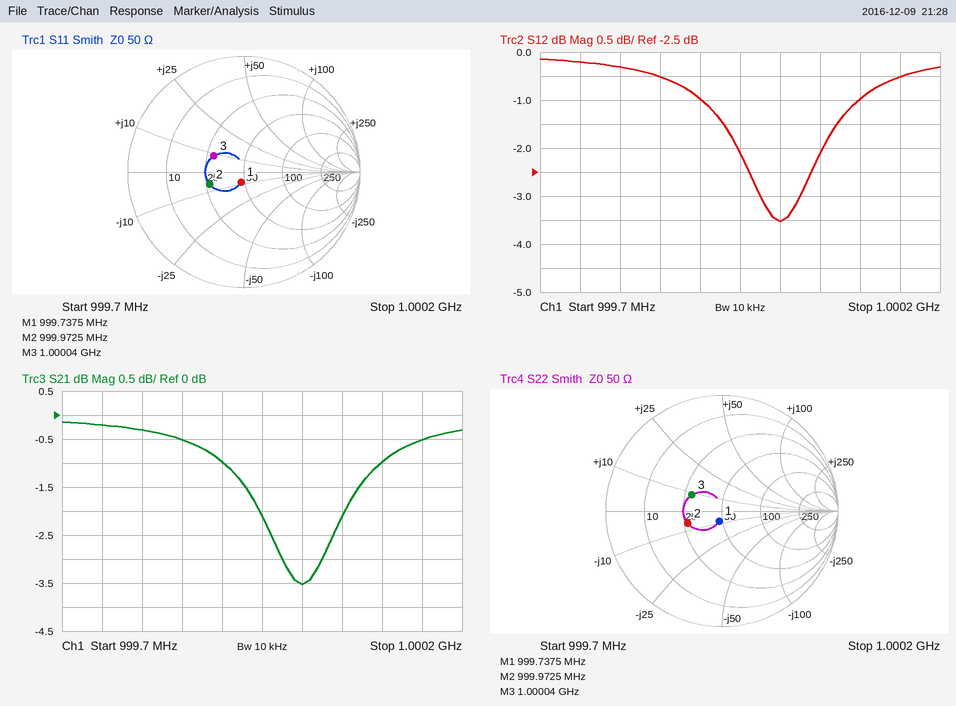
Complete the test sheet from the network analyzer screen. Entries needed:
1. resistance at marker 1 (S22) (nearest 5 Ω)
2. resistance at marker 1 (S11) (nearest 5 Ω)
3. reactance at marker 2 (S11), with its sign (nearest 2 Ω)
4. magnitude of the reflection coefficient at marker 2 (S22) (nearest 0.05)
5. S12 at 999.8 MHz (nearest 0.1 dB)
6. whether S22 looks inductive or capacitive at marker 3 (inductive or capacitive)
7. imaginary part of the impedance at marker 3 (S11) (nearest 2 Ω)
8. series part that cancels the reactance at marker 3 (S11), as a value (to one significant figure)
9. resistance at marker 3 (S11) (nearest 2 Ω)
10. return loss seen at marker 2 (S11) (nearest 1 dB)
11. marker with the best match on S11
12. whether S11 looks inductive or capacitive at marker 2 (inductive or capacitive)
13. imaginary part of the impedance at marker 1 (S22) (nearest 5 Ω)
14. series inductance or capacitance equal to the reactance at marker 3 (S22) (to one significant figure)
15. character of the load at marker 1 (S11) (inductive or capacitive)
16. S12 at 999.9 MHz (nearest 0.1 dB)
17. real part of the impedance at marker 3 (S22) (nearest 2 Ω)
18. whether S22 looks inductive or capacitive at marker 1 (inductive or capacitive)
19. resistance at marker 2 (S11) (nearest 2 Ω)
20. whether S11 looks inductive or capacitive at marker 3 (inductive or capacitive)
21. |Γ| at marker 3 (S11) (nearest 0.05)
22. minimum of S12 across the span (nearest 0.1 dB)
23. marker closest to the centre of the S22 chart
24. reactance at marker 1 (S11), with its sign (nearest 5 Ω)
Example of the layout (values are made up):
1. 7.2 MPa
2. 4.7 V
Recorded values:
1. 45 Ω
2. 45 Ω
3. -6 Ω
4. 0.30
5. -0.3 dB
6. inductive
7. +8 Ω
8. 20 pF
9. 28 Ω
10. 10 dB
11. marker 1
12. capacitive
13. -10 Ω
14. 1 nH
15. capacitive
16. -1.0 dB
17. 28 Ω
18. capacitive
19. 26 Ω
20. inductive
21. 0.30
22. -3.5 dB
23. marker 1
24. -10 Ω
